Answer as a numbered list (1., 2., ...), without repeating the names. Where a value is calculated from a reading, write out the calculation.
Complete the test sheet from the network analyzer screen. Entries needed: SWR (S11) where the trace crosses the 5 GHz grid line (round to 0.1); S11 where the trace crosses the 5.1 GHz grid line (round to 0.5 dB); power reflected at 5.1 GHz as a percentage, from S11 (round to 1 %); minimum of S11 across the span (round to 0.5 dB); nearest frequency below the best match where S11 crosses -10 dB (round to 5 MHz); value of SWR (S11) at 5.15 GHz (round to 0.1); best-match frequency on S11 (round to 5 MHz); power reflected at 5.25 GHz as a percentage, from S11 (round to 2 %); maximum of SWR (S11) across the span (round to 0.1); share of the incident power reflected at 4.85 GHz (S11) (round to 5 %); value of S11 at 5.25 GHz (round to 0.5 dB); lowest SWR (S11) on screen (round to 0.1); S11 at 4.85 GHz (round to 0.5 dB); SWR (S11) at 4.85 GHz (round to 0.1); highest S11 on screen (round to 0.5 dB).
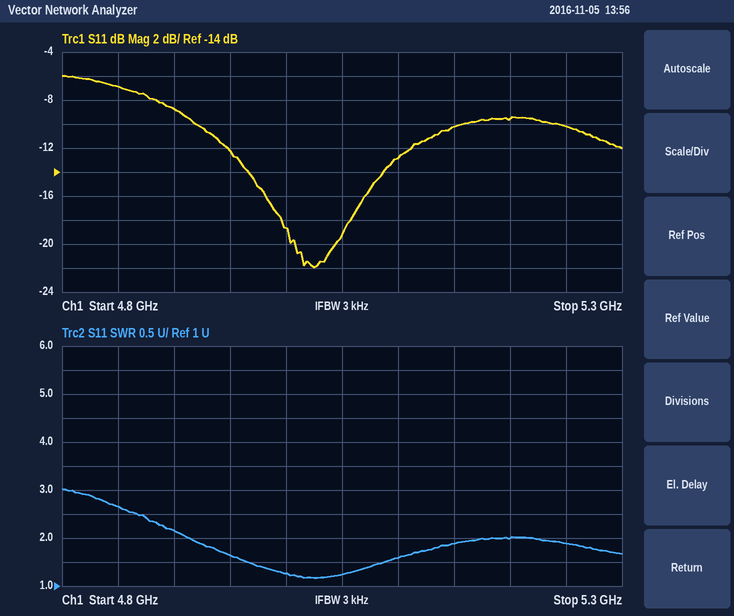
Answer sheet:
1. 1.3
2. -13.0 dB
3. 10^(-13/10) ≈ 5 %
4. -22.0 dB
5. 4.920 GHz
6. 1.9
7. 5.025 GHz
8. 10^(-10/10) ≈ 10 %
9. 3.0
10. 10^(-7/10) ≈ 20 %
11. -10.0 dB
12. 1.2
13. -7.0 dB
14. 2.7
15. -6.0 dB
